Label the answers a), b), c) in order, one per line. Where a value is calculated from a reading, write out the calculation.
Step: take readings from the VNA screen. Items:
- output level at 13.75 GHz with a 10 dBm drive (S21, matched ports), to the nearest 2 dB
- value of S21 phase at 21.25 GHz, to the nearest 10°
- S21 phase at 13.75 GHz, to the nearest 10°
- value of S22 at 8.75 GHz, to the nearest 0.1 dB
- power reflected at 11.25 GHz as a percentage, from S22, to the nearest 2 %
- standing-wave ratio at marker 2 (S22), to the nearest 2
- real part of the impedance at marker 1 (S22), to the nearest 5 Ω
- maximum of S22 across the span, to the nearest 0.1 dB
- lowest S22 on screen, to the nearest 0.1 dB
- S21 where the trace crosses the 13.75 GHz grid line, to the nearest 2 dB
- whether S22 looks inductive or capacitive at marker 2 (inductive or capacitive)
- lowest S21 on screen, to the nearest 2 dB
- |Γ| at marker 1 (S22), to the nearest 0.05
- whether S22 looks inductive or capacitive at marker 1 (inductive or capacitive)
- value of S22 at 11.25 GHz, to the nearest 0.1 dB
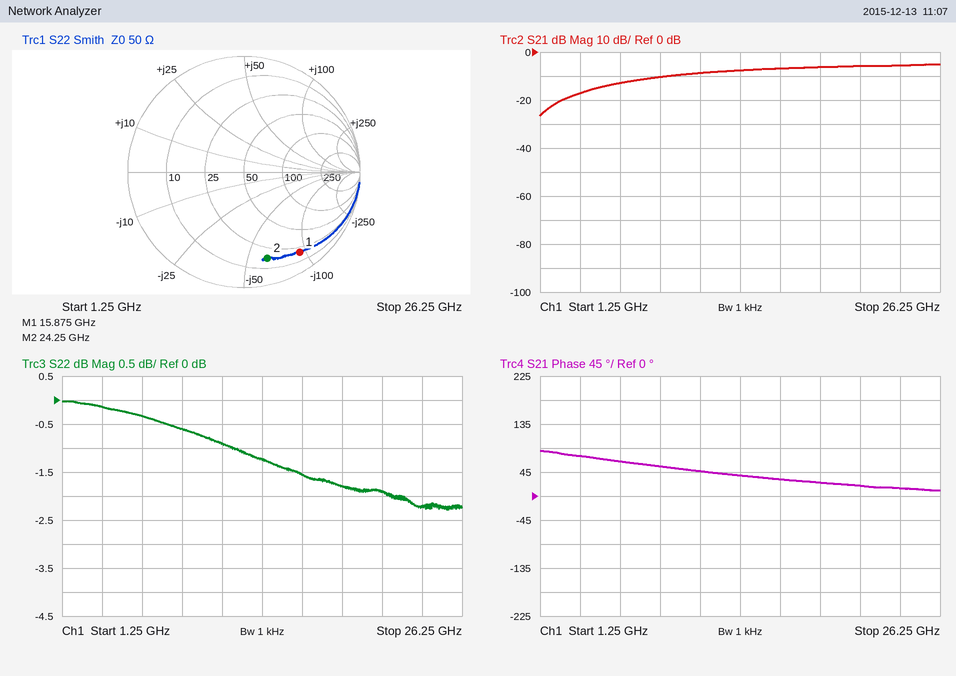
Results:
a) 10 dBm + (-8 dB) = 2 dBm
b) 20°
c) 40°
d) -0.6 dB
e) 10^(-0.9/10) ≈ 81.3 %, so 82 % to the nearest 2 %
f) 8
g) 20 Ω
h) 0.0 dB
i) -2.3 dB
j) -8 dB
k) capacitive
l) -26 dB
m) 0.85
n) capacitive
o) -0.9 dB
